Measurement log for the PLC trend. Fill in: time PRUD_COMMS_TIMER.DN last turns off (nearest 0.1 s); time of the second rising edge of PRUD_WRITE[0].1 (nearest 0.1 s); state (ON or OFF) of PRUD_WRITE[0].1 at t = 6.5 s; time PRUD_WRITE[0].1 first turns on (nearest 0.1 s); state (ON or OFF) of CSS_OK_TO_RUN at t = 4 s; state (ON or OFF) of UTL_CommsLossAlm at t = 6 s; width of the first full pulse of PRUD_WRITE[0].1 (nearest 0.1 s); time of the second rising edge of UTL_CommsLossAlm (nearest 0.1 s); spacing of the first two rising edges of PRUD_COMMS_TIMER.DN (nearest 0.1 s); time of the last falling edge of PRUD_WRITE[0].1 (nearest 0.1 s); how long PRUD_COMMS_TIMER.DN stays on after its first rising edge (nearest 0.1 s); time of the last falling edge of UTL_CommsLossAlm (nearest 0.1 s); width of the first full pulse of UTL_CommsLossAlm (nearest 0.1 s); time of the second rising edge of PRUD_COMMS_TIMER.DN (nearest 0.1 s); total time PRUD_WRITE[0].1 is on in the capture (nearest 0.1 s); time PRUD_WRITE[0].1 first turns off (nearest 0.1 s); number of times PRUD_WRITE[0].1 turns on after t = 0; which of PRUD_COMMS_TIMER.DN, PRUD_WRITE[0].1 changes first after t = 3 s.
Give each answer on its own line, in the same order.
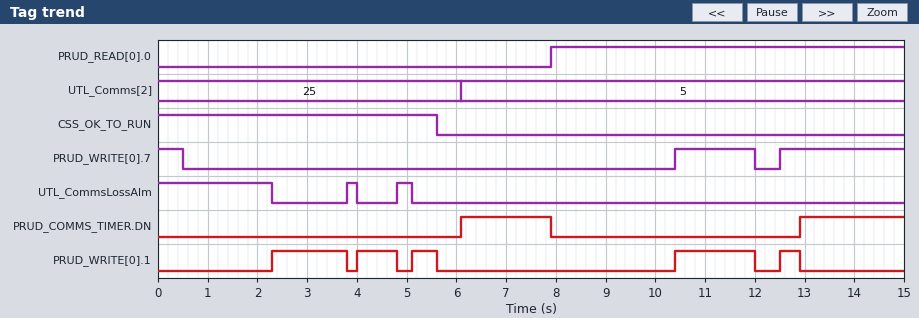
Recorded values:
7.9 s
4.0 s
OFF
2.3 s
ON
OFF
1.5 s
4.8 s
6.8 s
12.9 s
1.8 s
5.1 s
0.2 s
12.9 s
4.8 s
3.8 s
5
PRUD_WRITE[0].1
